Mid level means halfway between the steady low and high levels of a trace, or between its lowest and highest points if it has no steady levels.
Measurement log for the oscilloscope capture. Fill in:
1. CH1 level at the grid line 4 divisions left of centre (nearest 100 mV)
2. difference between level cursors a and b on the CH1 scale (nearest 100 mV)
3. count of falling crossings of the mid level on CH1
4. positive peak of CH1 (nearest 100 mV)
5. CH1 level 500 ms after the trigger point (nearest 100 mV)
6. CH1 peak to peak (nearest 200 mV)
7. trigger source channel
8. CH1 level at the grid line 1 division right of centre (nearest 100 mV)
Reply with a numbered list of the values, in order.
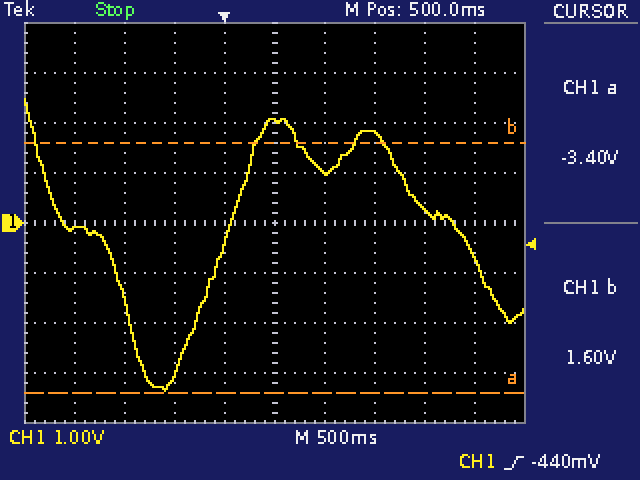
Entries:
1. -100 mV
2. 5.0 V
3. 2
4. 2.5 V
5. 2.0 V
6. 5.8 V
7. CH1
8. 1.0 V
